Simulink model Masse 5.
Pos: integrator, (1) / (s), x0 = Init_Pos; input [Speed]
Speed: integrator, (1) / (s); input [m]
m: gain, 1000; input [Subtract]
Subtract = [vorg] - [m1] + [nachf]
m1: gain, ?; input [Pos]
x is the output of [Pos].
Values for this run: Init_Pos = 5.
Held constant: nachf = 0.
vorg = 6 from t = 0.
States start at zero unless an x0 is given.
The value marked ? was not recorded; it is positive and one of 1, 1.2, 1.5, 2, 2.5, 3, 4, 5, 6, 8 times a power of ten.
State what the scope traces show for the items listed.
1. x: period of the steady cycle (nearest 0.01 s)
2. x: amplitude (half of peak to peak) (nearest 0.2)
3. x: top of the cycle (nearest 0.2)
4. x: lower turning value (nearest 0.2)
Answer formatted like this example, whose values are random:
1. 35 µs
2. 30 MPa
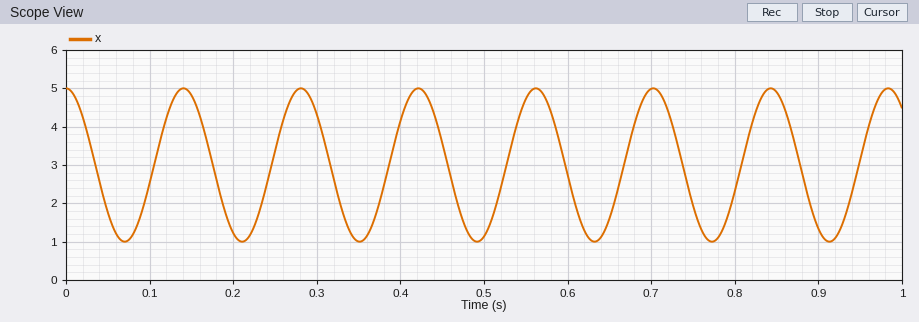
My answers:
1. 0.14 s
2. 2.0
3. 5.0
4. 1.0
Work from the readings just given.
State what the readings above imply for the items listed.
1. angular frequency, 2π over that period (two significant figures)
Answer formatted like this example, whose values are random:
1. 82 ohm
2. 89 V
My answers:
1. 45 rad/s
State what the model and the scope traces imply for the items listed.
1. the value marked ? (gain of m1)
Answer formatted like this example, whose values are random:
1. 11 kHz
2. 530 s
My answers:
1. 2
